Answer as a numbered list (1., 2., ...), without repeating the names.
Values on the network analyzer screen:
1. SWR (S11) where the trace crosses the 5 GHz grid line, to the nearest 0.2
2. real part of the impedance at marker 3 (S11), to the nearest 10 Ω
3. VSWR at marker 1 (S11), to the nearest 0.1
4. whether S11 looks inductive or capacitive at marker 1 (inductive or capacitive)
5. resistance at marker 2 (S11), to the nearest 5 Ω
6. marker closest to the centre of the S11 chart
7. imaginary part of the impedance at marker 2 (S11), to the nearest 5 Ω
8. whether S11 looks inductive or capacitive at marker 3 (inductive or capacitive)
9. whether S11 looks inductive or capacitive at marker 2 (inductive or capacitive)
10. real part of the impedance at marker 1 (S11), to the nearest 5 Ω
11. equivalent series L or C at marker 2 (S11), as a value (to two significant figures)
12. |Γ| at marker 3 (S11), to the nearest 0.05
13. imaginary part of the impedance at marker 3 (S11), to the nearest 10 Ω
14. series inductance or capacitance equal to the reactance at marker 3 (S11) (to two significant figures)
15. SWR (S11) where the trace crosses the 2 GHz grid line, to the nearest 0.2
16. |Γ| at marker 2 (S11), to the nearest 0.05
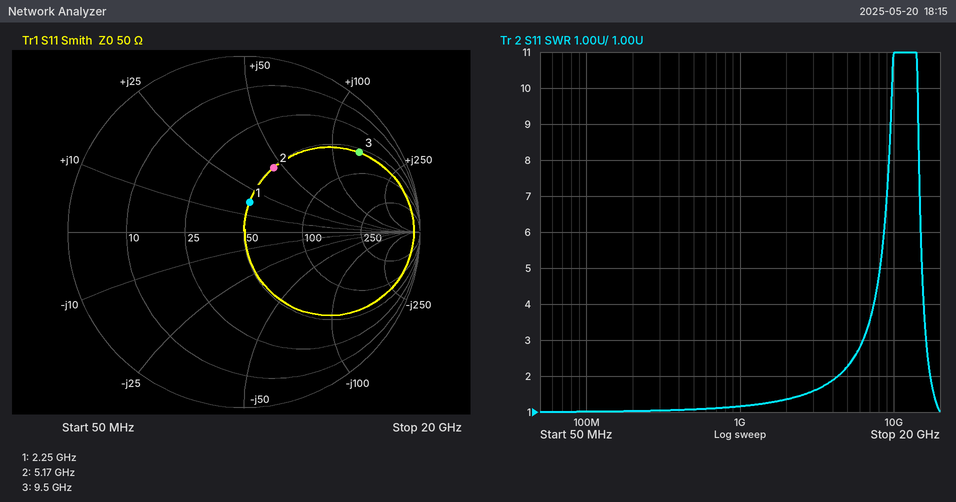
1. 2.2
2. 60 Ω
3. 1.4
4. inductive
5. 50 Ω
6. marker 1
7. +45 Ω
8. inductive
9. inductive
10. 50 Ω
11. 1.4 nH
12. 0.80
13. +140 Ω
14. 2.3 nH
15. 1.4
16. 0.40
